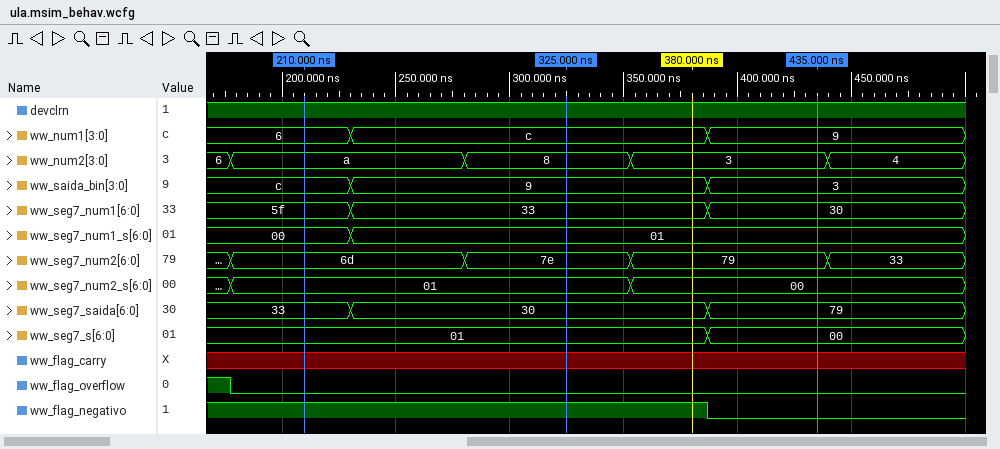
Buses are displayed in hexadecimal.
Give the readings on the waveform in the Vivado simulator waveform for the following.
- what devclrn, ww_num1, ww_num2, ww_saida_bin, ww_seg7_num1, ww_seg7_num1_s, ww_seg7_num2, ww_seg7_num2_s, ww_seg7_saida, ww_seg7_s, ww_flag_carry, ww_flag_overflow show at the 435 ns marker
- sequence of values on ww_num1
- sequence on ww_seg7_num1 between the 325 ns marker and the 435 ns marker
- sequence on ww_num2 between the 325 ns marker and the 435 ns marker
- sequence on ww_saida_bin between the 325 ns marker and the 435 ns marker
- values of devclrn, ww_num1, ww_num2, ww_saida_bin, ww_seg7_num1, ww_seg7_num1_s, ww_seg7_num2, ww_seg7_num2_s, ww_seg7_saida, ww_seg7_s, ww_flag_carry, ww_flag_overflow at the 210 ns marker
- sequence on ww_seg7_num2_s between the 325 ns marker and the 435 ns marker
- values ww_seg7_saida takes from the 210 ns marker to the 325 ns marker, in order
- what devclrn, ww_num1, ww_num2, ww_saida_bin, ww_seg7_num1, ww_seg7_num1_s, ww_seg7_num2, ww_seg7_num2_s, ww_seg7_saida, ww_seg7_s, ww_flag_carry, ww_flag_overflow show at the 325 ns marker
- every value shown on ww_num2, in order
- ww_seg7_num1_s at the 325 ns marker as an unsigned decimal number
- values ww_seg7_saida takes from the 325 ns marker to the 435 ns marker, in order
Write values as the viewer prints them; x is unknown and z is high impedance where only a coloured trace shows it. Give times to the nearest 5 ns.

devclrn=1, ww_num1=9, ww_num2=3, ww_saida_bin=3, ww_seg7_num1=30, ww_seg7_num1_s=01, ww_seg7_num2=79, ww_seg7_num2_s=00, ww_seg7_saida=79, ww_seg7_s=00, ww_flag_carry=x, ww_flag_overflow=0
6, c, 9
33, 30
8, 3
9, 3
devclrn=1, ww_num1=6, ww_num2=a, ww_saida_bin=c, ww_seg7_num1=5f, ww_seg7_num1_s=00, ww_seg7_num2=6d, ww_seg7_num2_s=01, ww_seg7_saida=33, ww_seg7_s=01, ww_flag_carry=x, ww_flag_overflow=0
01, 00
33, 30
devclrn=1, ww_num1=c, ww_num2=8, ww_saida_bin=9, ww_seg7_num1=33, ww_seg7_num1_s=01, ww_seg7_num2=7e, ww_seg7_num2_s=01, ww_seg7_saida=30, ww_seg7_s=01, ww_flag_carry=x, ww_flag_overflow=0
6, a, 8, 3, 4
1
30, 79
